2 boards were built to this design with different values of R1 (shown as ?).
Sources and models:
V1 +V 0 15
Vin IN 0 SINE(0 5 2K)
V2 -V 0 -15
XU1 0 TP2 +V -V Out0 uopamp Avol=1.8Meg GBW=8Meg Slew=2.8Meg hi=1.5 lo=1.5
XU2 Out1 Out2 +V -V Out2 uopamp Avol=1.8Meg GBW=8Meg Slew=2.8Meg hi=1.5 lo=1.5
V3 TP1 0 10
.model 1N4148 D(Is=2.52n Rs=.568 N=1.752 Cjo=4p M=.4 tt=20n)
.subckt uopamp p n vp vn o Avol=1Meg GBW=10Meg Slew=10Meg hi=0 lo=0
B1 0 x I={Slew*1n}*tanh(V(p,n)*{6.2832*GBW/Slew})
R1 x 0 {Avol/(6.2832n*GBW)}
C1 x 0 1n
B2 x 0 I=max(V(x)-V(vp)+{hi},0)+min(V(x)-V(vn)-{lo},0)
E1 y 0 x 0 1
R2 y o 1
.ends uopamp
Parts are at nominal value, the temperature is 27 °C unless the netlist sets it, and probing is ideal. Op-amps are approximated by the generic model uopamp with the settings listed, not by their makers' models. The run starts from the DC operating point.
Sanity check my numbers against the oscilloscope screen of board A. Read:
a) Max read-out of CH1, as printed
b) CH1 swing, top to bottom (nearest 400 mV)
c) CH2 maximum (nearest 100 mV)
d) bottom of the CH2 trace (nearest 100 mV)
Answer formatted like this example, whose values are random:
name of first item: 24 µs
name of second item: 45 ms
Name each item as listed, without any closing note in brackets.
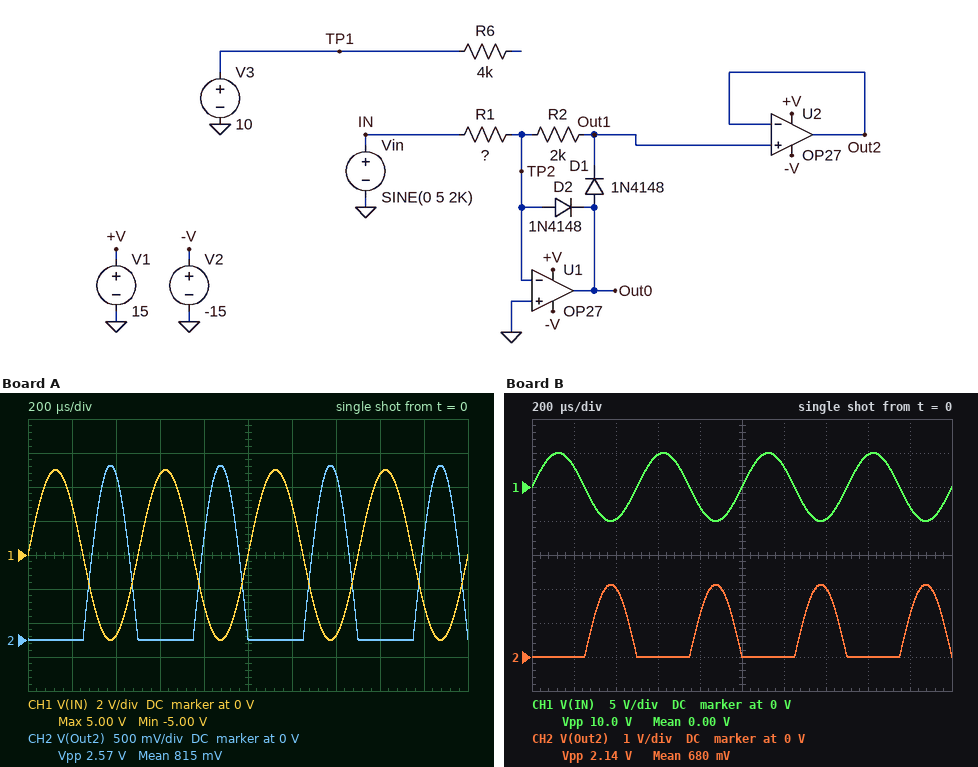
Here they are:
Max read-out of CH1, as printed: 5.00 V
CH1 swing, top to bottom: 10.0 V
CH2 maximum: 2.6 V
bottom of the CH2 trace: 0 V
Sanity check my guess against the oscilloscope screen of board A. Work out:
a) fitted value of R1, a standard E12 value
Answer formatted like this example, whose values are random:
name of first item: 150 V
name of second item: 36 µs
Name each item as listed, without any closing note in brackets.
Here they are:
fitted value of R1, a standard E12 value: 3.9 kΩ
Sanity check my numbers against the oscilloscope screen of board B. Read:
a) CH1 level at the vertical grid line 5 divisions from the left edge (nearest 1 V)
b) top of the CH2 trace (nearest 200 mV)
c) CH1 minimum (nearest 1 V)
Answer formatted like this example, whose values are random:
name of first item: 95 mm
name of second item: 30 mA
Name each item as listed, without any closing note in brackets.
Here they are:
CH1 level at the vertical grid line 5 divisions from the left edge: 0 V
top of the CH2 trace: 2.2 V
CH1 minimum: -5 V
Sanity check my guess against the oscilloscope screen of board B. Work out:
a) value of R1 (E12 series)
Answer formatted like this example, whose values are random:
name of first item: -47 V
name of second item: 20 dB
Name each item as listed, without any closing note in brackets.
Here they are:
value of R1: 4.7 kΩ
